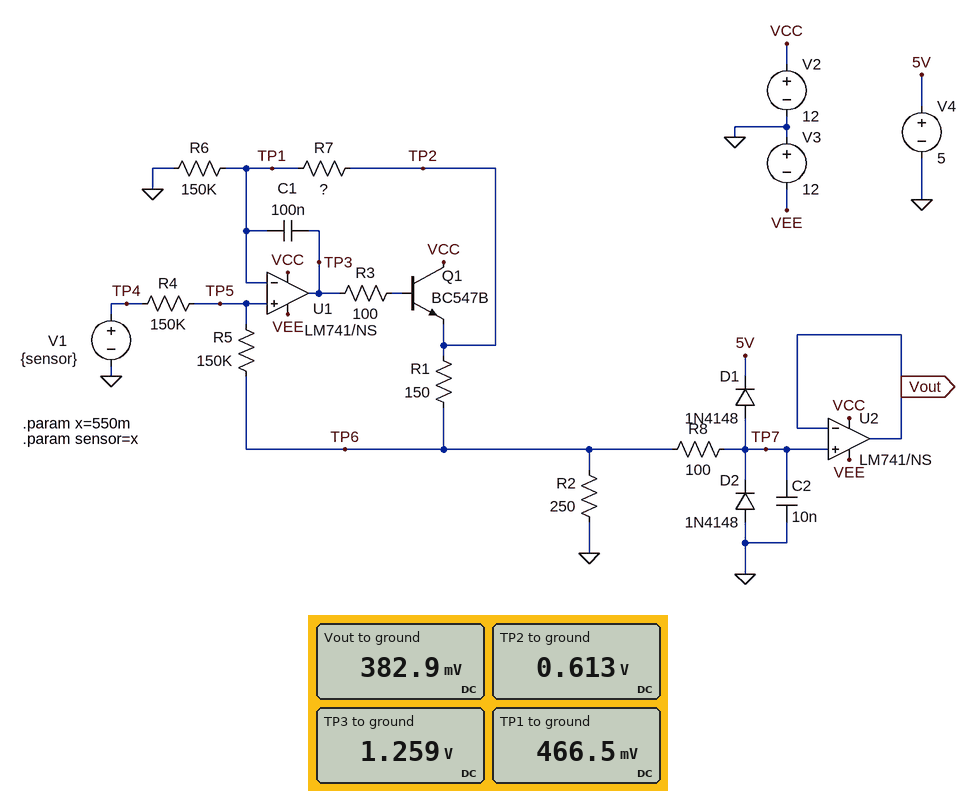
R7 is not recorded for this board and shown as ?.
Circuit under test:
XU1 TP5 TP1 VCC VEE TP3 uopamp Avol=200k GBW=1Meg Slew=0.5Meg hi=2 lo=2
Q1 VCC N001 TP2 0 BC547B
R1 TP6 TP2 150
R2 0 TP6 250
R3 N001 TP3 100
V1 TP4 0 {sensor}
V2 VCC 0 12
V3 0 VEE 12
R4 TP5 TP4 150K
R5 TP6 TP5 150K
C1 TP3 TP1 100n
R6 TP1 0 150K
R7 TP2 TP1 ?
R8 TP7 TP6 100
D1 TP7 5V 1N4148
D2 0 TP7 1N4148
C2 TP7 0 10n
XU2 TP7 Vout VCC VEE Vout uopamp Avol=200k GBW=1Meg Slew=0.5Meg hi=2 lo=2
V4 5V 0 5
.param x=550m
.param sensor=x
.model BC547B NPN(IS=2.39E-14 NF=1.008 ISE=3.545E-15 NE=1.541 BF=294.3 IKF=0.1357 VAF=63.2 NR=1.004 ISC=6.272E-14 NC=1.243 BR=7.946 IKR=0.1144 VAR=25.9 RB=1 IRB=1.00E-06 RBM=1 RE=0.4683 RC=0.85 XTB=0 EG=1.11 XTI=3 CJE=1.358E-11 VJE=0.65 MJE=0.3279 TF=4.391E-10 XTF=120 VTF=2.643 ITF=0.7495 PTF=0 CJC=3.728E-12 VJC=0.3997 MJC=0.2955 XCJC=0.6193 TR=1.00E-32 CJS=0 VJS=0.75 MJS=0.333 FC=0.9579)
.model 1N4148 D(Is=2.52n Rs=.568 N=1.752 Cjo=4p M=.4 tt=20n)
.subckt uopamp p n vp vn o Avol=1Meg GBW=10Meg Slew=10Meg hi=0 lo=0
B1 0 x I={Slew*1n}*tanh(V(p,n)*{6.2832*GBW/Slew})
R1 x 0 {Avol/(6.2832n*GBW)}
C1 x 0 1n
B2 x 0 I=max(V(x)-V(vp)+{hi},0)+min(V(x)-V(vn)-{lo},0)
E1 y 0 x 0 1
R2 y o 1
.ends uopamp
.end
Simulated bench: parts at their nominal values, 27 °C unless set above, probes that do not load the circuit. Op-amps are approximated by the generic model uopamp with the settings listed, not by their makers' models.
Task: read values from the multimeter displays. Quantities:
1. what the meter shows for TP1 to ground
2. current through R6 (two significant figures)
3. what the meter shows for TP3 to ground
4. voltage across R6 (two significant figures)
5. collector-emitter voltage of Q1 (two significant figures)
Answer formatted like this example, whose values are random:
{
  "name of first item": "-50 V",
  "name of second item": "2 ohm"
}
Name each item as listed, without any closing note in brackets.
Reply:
{
  "what the meter shows for TP1 to ground": "466.5 mV",
  "current through R6": "3.1 µA",
  "what the meter shows for TP3 to ground": "1.259 V",
  "voltage across R6": "470 mV",
  "collector-emitter voltage of Q1": "11 V"
}
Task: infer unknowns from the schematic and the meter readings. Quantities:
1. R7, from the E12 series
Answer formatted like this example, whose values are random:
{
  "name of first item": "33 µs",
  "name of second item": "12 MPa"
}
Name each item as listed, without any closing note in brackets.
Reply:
{
  "R7, from the E12 series": "47 kΩ"
}
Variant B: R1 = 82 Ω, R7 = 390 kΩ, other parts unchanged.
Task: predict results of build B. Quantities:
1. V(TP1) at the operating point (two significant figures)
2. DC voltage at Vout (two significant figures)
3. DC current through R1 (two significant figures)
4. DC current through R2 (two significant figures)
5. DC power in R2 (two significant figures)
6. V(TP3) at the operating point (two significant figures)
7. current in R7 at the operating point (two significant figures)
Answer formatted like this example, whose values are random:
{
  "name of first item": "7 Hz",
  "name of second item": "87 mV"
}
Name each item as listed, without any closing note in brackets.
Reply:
{
  "V(TP1) at the operating point": "2.6 V",
  "DC voltage at Vout": "5.7 V",
  "DC current through R1": "34 mA",
  "DC current through R2": "26 mA",
  "DC power in R2": "170 mW",
  "V(TP3) at the operating point": "10 V",
  "current in R7 at the operating point": "17 µA"
}
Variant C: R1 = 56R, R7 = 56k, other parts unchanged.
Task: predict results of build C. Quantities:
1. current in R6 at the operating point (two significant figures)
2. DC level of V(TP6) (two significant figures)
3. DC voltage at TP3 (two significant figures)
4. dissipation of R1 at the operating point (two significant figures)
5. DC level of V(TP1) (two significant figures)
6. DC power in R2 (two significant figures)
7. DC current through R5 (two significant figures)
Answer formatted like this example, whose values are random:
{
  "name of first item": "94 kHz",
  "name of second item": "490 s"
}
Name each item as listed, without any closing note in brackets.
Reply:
{
  "current in R6 at the operating point": "4.2 µA",
  "DC level of V(TP6)": "700 mV",
  "DC voltage at TP3": "1.5 V",
  "dissipation of R1 at the operating point": "440 µW",
  "DC level of V(TP1)": "630 mV",
  "DC power in R2": "2.0 mW",
  "DC current through R5": "510 nA"
}
